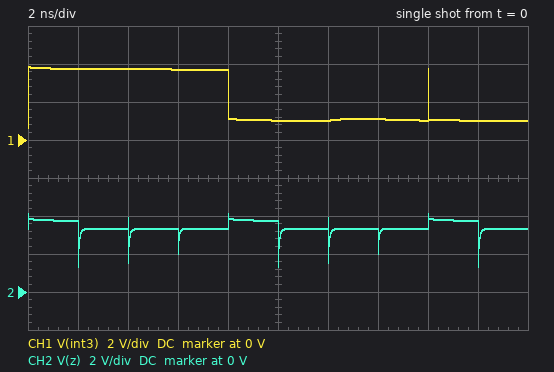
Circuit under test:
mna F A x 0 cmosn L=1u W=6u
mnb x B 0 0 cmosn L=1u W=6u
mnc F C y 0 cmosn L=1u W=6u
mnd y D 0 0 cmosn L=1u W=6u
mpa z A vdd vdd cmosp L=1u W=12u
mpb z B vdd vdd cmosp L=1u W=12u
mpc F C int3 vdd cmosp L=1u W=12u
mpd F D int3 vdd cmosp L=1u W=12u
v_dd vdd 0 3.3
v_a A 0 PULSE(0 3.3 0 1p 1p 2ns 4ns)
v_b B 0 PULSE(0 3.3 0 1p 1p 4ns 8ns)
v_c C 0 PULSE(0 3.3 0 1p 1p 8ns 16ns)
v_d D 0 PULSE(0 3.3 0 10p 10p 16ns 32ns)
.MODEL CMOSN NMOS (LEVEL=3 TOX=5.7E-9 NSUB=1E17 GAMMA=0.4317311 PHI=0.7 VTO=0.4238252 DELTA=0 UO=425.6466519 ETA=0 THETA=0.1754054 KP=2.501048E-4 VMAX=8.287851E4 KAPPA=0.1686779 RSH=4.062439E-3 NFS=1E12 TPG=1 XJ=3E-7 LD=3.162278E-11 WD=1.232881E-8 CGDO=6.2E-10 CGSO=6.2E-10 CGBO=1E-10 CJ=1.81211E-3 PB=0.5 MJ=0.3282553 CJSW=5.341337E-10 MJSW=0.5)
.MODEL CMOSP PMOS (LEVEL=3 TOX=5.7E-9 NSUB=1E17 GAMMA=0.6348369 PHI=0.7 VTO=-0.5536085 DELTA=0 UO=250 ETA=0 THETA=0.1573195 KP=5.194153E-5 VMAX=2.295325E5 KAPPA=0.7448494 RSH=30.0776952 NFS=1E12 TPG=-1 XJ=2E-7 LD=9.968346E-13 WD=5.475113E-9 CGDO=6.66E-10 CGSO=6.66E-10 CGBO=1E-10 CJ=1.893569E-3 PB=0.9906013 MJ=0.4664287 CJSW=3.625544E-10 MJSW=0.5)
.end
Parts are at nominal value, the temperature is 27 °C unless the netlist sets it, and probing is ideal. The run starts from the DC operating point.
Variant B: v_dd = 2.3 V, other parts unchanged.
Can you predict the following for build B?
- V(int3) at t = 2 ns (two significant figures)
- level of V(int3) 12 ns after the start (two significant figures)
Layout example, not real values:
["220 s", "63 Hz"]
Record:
["2.7 V", "780 mV"]
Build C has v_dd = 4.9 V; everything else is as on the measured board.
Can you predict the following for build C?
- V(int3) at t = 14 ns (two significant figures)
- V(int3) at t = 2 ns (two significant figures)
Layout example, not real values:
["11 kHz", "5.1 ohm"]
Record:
["1.2 V", "4.1 V"]
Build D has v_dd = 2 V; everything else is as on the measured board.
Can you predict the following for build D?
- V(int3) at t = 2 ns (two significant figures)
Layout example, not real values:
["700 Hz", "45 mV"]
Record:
["2.4 V"]
